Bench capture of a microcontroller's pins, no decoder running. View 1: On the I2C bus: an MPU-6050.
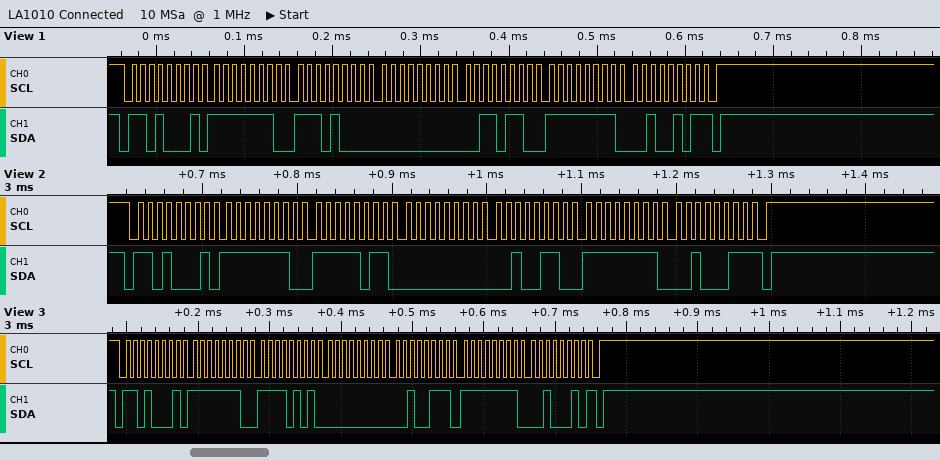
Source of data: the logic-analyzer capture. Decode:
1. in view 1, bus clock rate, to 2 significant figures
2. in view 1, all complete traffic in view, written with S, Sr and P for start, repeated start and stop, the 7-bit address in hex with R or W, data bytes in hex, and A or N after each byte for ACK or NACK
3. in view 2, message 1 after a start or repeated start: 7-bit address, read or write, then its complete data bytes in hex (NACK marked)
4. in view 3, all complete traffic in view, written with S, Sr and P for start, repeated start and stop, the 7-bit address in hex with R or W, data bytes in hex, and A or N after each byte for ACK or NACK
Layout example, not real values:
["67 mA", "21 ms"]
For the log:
["100 kHz", "S 68R A FE A E8 A 00 A 36 A FF A 25 N P", "0x68 read: FE FB 00 26 FF 23 NACK", "S 68R A FE A F5 A 00 A 27 A FF A 22 N P"]
